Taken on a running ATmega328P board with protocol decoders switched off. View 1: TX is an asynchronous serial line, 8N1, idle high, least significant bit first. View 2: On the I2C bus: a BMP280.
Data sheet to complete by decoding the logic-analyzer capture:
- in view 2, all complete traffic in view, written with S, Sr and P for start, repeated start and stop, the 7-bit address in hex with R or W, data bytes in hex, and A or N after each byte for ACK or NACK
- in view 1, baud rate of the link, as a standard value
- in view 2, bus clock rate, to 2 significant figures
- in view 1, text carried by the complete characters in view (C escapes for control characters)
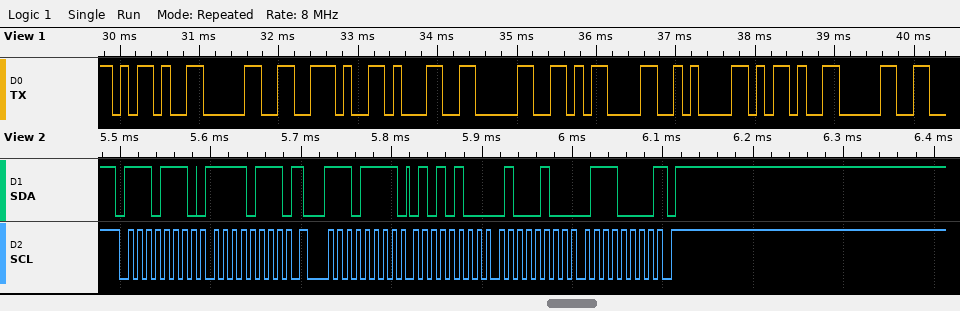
S 77W A F7 A Sr 77R A 54 A 44 A 70 N P
9600 baud
100 kHz
"-0.10\r\n-0"
